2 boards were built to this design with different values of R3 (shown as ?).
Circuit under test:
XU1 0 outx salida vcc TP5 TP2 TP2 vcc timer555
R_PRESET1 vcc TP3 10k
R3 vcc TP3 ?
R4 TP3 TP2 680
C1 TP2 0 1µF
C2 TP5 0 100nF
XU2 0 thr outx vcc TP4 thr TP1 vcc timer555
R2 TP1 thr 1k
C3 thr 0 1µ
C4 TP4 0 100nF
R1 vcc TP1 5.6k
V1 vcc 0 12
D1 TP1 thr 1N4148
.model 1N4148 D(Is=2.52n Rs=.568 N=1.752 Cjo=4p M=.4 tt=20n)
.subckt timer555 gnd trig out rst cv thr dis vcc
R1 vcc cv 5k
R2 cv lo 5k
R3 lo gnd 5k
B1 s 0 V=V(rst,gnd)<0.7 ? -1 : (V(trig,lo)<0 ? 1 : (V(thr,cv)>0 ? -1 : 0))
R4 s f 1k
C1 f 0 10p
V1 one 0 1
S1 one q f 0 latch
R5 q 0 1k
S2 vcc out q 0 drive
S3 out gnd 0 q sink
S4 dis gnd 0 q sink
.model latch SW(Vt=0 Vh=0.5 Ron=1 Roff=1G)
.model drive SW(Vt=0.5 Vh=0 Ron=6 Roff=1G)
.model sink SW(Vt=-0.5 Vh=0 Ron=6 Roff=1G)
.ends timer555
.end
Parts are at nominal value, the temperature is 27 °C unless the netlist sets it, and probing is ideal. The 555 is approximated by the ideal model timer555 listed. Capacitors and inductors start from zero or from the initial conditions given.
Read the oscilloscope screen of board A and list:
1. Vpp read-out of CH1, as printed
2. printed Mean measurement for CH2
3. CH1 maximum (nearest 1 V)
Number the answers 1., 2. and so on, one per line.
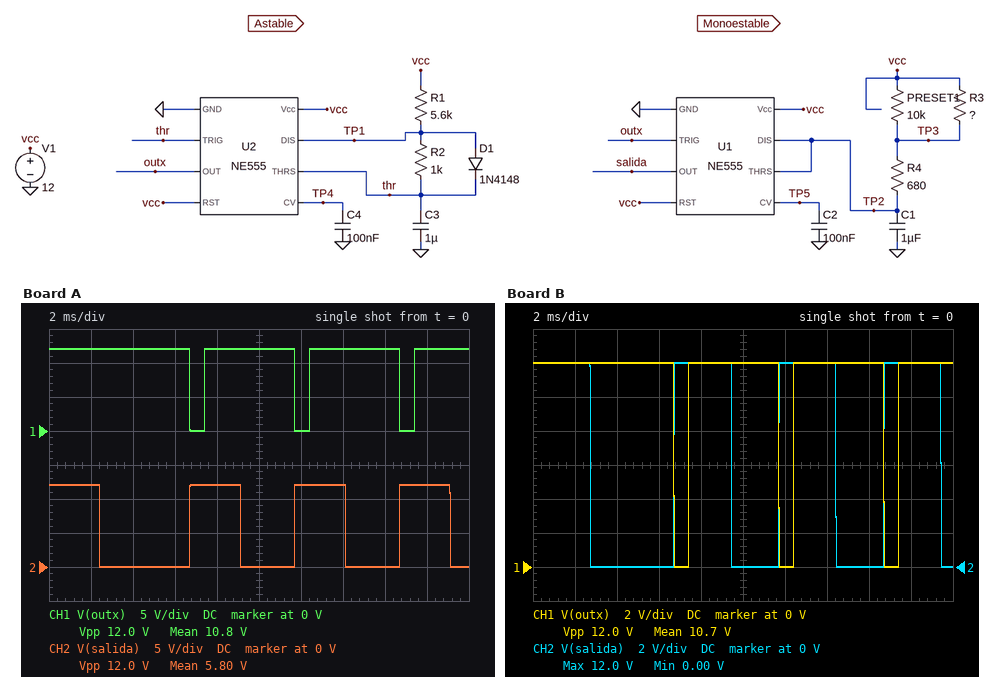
1. 12.0 V
2. 5.80 V
3. 12 V
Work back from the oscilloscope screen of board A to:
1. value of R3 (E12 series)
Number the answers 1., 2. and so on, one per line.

1. 1.8 kΩ
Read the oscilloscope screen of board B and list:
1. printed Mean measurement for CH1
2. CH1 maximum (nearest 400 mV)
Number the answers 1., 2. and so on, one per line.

1. 10.7 V
2. 12.0 V
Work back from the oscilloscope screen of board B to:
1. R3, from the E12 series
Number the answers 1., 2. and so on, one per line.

1. 2.2 kΩ
